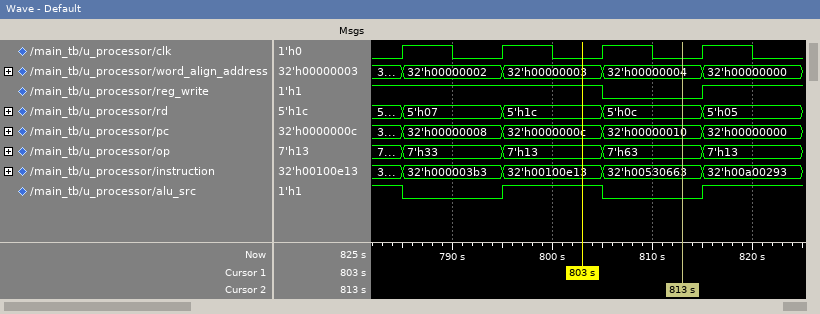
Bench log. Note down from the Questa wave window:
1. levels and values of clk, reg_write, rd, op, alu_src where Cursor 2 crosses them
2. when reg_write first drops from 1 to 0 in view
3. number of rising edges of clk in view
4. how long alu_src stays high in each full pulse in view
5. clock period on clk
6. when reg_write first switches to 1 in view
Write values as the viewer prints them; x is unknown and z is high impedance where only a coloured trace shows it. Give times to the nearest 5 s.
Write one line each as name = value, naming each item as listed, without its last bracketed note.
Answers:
levels and values of clk, reg_write, rd, op, alu_src where Cursor 2 crosses them = clk=0, reg_write=0, rd=5'h0c, op=7'h63, alu_src=0
when reg_write first drops from 1 to 0 in view = 805 s
number of rising edges of clk in view = 4
how long alu_src stays high in each full pulse in view = 10 s
clock period on clk = 10 s
when reg_write first switches to 1 in view = 815 s
